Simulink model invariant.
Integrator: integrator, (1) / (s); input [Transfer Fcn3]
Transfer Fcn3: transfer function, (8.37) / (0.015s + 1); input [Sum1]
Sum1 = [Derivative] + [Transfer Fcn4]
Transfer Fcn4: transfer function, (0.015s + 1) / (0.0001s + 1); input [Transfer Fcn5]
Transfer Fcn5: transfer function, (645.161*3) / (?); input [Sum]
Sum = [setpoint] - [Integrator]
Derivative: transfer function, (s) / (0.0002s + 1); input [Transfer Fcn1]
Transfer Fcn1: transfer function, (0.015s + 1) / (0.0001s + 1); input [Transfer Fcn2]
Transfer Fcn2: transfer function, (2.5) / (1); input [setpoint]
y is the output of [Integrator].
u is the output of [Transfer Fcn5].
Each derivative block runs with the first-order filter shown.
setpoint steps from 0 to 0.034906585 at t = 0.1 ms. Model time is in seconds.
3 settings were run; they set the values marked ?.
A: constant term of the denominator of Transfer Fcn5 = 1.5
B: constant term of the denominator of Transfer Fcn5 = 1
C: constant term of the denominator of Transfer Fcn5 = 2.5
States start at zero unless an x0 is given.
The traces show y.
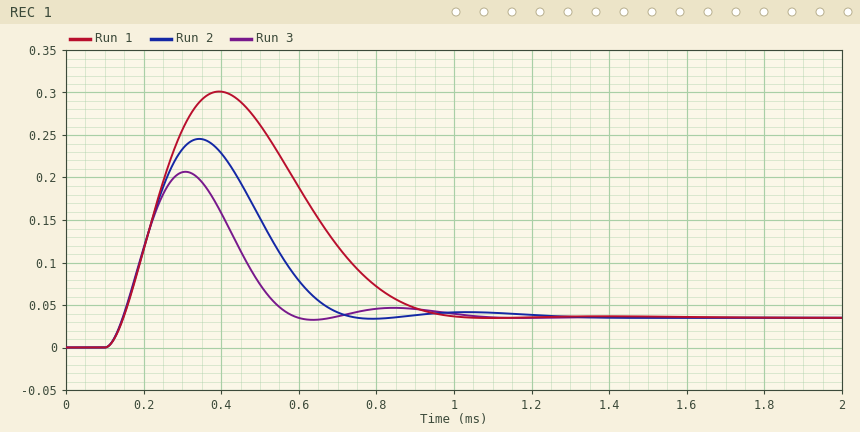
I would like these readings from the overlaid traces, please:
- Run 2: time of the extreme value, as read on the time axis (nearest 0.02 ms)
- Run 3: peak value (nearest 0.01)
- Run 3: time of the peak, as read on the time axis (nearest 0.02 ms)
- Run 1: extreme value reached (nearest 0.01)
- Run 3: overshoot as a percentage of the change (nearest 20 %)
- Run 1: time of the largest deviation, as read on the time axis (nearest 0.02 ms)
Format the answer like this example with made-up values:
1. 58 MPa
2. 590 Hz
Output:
1. 0.34 ms
2. 0.21
3. 0.30 ms
4. 0.30
5. 500 %
6. 0.40 ms
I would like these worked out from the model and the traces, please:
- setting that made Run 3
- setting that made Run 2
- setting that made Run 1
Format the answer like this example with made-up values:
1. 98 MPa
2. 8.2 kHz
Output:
1. B
2. A
3. C
